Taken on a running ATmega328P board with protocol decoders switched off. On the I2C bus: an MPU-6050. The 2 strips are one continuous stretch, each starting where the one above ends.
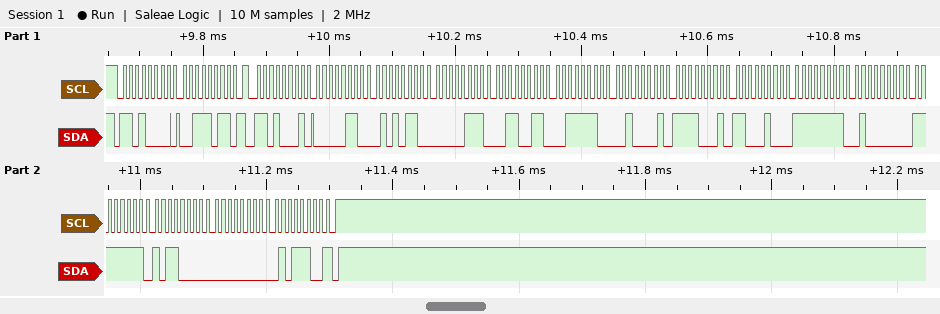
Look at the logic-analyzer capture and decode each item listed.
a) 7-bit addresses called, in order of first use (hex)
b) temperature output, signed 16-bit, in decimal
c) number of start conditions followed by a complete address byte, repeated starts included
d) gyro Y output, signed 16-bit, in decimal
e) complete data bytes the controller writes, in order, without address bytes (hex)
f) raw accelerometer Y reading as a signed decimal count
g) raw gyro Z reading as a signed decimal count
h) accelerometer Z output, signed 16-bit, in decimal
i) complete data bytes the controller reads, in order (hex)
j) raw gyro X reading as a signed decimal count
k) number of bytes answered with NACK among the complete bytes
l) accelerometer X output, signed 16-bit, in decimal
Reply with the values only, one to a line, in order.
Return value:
0x68
-3644
2
-80
3B
1843
92
15905
06 56 07 33 3E 21 F1 C4 FF 40 FF B0 00 5C
-192
1
1622
